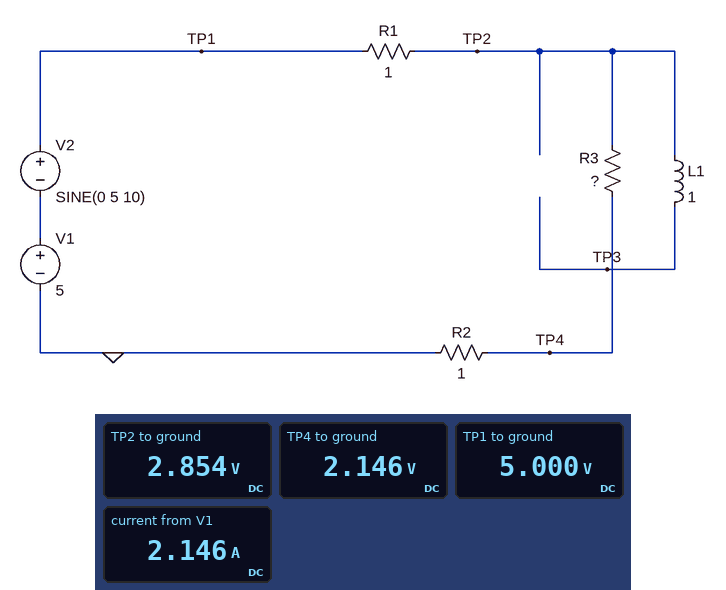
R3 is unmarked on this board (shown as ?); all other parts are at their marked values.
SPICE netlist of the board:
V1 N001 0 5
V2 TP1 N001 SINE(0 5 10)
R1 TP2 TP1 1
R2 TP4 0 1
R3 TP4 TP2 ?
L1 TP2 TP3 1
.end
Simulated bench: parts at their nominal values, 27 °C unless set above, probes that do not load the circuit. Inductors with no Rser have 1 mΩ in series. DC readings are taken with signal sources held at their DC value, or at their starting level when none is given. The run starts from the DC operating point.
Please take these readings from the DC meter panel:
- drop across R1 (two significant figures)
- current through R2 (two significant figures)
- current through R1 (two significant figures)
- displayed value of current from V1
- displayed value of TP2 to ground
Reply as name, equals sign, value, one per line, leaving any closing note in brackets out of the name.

drop across R1 = 2.1 V
current through R2 = 2.1 A
current through R1 = 2.1 A
displayed value of current from V1 = 2.146 A
displayed value of TP2 to ground = 2.854 V
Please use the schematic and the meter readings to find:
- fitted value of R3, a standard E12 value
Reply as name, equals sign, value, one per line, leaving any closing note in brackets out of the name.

fitted value of R3, a standard E12 value = 0.33 Ω
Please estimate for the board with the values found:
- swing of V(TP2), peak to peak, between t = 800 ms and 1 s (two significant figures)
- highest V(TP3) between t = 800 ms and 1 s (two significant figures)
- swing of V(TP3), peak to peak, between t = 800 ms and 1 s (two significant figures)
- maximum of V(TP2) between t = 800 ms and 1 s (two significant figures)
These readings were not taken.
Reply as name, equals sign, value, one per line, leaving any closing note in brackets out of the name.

swing of V(TP2), peak to peak, between t = 800 ms and 1 s = 5.7 V
highest V(TP3) between t = 800 ms and 1 s = 5.7 V
swing of V(TP3), peak to peak, between t = 800 ms and 1 s = 5.7 V
maximum of V(TP2) between t = 800 ms and 1 s = 5.7 V
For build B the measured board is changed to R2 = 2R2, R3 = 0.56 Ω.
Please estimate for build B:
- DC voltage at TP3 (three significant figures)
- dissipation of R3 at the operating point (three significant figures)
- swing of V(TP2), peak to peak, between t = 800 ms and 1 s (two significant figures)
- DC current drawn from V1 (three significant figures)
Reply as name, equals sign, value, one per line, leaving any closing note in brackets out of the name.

DC voltage at TP3 = 3.67 V
dissipation of R3 at the operating point = 990 mW
swing of V(TP2), peak to peak, between t = 800 ms and 1 s = 7.3 V
DC current drawn from V1 = 1.33 A
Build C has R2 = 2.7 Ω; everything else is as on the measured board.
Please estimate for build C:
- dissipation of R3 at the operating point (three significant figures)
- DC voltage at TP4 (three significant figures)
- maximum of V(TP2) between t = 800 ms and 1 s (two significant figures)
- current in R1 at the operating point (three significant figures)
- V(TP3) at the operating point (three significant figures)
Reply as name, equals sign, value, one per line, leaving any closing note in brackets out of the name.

dissipation of R3 at the operating point = 508 mW
DC voltage at TP4 = 3.35 V
maximum of V(TP2) between t = 800 ms and 1 s = 7.5 V
current in R1 at the operating point = 1.24 A
V(TP3) at the operating point = 3.76 V
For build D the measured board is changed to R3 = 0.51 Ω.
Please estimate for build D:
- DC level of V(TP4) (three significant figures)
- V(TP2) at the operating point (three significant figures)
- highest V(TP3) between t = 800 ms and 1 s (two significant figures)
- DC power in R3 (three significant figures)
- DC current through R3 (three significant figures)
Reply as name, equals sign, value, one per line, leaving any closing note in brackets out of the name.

DC level of V(TP4) = 1.99 V
V(TP2) at the operating point = 3.01 V
highest V(TP3) between t = 800 ms and 1 s = 6.0 V
DC power in R3 = 2.02 W
DC current through R3 = 1.99 A
